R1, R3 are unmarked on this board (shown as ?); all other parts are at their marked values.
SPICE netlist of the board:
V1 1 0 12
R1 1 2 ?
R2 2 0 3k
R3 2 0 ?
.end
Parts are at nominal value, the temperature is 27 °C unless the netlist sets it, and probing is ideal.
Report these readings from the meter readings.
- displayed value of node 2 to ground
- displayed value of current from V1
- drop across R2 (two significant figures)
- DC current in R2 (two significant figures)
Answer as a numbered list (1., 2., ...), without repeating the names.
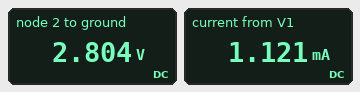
1. 2.804 V
2. 1.121 mA
3. 2.8 V
4. 930 µA
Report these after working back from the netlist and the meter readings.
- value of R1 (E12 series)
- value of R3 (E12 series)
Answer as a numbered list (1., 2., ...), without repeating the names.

1. 8.2 kΩ
2. 15 kΩ
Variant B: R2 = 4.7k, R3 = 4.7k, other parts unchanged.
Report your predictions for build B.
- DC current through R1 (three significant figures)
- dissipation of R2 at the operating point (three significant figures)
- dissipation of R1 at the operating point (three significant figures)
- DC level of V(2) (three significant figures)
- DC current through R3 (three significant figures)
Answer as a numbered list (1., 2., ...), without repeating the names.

1. 1.14 mA
2. 1.52 mW
3. 10.6 mW
4. 2.67 V
5. 569 µA
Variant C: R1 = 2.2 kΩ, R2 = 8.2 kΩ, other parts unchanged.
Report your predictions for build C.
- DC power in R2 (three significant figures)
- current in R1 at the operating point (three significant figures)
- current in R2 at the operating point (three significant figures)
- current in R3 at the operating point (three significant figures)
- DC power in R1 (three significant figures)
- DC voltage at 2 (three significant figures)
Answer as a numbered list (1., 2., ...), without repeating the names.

1. 8.77 mW
2. 1.60 mA
3. 1.03 mA
4. 565 µA
5. 5.63 mW
6. 8.48 V
